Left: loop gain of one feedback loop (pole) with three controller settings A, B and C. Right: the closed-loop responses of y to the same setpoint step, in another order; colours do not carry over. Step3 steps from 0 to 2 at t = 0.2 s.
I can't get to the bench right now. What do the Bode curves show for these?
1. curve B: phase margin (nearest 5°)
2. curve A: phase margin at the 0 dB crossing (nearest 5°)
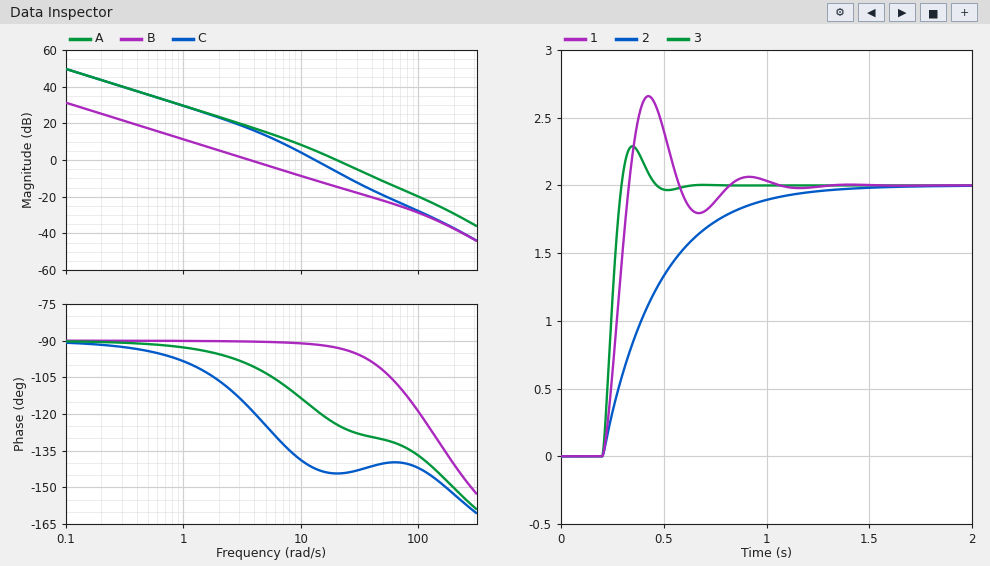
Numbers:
90°
55°
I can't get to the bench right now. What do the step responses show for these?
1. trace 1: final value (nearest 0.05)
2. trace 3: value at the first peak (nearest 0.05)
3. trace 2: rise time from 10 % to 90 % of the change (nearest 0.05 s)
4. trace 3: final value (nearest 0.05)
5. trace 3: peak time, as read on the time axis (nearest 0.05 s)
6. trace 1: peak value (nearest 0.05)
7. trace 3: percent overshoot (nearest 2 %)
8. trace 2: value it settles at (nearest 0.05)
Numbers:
2.00
2.30
0.60 s
2.00
0.35 s
2.65
14 %
2.00
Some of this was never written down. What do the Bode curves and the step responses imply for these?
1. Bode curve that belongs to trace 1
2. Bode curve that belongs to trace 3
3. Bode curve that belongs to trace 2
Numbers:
C
A
B
